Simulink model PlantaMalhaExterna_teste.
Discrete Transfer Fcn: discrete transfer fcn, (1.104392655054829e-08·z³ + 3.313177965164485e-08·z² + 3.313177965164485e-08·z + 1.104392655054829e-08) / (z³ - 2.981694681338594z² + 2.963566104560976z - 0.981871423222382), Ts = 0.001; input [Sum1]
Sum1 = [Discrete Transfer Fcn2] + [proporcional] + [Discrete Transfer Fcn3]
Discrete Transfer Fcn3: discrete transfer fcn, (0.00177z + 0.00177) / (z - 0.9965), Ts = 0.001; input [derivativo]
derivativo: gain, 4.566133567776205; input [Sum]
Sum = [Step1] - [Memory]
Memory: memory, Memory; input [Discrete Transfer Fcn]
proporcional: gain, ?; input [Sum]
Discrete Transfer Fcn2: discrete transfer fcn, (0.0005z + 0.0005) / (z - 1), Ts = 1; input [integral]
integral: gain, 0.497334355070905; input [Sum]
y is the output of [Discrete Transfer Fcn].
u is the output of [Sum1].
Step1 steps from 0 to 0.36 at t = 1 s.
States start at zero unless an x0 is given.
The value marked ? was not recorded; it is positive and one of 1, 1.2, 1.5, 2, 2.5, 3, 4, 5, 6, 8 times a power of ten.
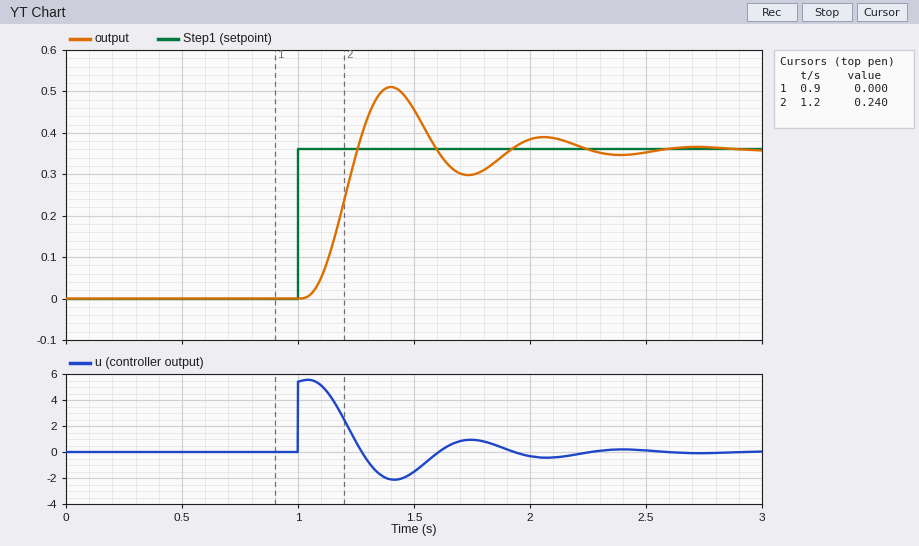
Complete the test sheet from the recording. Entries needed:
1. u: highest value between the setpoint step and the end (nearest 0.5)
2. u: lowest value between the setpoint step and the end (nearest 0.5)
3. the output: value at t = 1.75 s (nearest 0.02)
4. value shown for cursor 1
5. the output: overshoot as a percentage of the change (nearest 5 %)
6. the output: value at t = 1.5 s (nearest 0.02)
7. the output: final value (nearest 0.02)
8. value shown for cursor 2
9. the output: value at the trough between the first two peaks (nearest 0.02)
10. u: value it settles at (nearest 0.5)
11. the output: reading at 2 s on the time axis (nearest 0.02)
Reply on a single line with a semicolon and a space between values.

5.5; -2.0; 0.30; 0.000; 40 %; 0.46; 0.36; 0.240; 0.30; 0.0; 0.38
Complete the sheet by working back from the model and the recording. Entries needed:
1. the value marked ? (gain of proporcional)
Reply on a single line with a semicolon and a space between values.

15
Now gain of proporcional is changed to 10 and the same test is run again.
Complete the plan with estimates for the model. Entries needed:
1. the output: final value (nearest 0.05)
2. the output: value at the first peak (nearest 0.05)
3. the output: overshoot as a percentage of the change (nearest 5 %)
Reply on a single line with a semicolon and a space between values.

0.35; 0.45; 30 %
